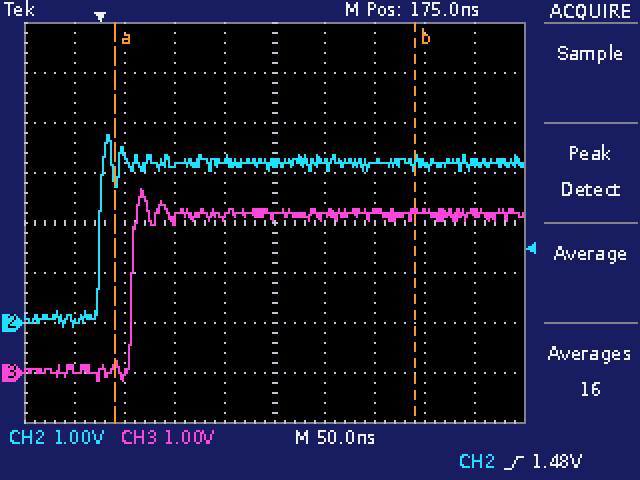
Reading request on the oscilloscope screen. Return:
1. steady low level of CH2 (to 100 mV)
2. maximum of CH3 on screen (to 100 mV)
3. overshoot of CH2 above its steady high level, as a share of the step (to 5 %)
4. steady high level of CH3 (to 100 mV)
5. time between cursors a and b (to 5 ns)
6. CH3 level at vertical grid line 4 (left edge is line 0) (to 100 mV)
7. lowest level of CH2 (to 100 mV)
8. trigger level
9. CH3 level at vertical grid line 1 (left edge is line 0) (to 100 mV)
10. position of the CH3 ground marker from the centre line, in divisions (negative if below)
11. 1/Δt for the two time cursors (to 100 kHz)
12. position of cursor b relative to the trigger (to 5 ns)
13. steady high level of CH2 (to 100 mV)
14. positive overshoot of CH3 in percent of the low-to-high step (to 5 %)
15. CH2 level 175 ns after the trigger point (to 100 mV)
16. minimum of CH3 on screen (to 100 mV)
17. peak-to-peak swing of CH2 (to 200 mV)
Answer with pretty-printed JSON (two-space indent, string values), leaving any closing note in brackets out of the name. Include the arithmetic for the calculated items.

{
  "steady low level of CH2": "100 mV",
  "maximum of CH3 on screen": "3.7 V",
  "overshoot of CH2 above its steady high level, as a share of the step": "20 %",
  "steady high level of CH3": "3.2 V",
  "time between cursors a and b": "300 ns",
  "CH3 level at vertical grid line 4 (left edge is line 0)": "3.1 V",
  "lowest level of CH2": "-100 mV",
  "trigger level": "1.48 V",
  "CH3 level at vertical grid line 1 (left edge is line 0)": "100 mV",
  "position of the CH3 ground marker from the centre line, in divisions": "-3.0 div",
  "1/Δt for the two time cursors": "1 / 300 ns ≈ 3.3 MHz",
  "position of cursor b relative to the trigger": "+315 ns",
  "steady high level of CH2": "3.2 V",
  "positive overshoot of CH3 in percent of the low-to-high step": "15 %",
  "CH2 level 175 ns after the trigger point": "3.2 V",
  "minimum of CH3 on screen": "-200 mV",
  "peak-to-peak swing of CH2": "3.8 V"
}
